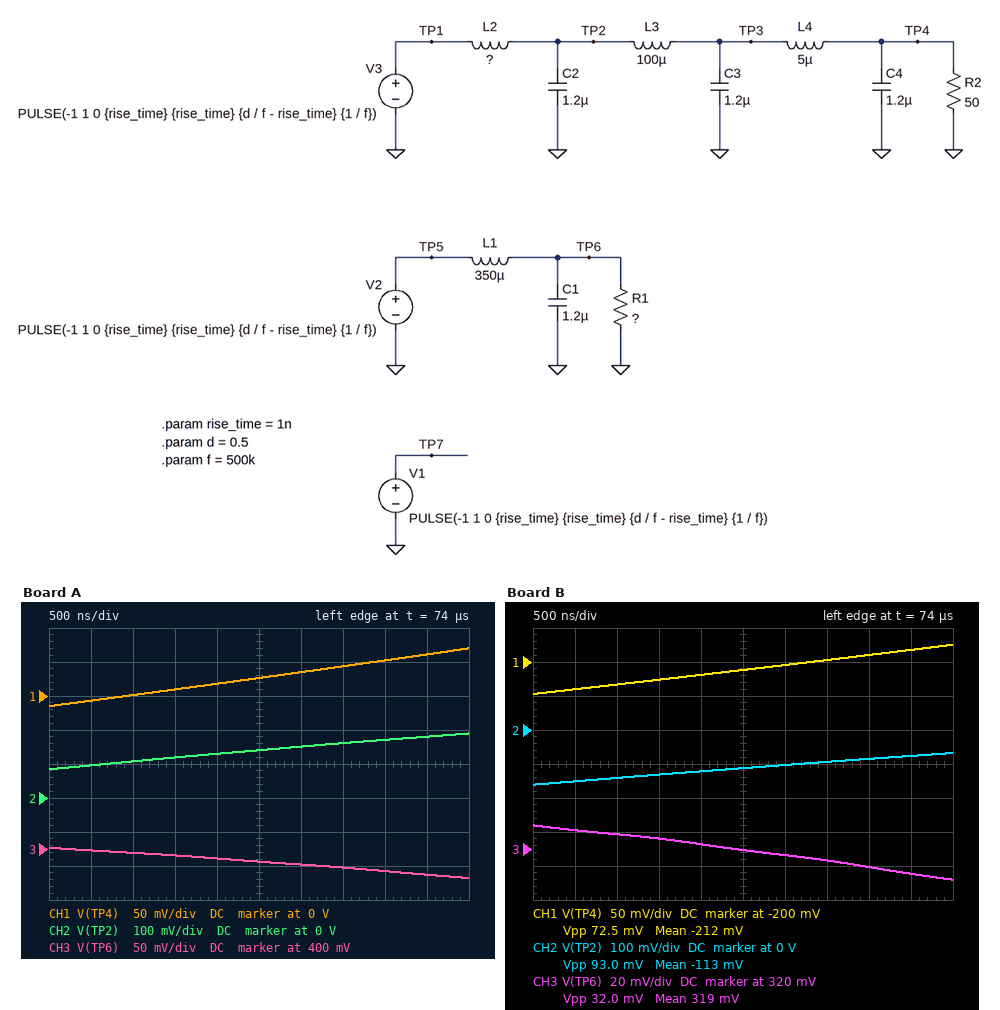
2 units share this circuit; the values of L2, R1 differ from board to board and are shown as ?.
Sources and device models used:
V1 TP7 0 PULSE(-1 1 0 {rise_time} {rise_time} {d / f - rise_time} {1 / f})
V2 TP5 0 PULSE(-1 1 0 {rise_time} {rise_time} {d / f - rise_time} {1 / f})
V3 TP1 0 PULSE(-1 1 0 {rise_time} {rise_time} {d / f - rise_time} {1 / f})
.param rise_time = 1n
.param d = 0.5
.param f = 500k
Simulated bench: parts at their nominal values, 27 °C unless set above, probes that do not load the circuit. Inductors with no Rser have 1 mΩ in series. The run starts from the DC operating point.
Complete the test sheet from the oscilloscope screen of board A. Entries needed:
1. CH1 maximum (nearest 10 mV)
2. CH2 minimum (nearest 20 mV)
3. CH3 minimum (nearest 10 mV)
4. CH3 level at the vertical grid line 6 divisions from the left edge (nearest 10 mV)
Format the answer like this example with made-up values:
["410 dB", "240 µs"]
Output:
["70 mV", "80 mV", "360 mV", "380 mV"]
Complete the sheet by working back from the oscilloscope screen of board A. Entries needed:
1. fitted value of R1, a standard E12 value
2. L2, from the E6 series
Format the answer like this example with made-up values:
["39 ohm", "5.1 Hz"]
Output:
["33 Ω", "470 µH"]
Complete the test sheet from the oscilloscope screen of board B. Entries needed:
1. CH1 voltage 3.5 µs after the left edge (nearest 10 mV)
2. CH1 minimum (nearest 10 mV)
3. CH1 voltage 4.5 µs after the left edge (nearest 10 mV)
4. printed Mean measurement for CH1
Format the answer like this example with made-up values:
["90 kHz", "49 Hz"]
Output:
["-200 mV", "-250 mV", "-180 mV", "-212 mV"]
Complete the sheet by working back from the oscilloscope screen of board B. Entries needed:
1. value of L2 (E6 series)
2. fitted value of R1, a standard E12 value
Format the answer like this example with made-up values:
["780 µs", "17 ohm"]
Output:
["680 µH", "27 Ω"]
